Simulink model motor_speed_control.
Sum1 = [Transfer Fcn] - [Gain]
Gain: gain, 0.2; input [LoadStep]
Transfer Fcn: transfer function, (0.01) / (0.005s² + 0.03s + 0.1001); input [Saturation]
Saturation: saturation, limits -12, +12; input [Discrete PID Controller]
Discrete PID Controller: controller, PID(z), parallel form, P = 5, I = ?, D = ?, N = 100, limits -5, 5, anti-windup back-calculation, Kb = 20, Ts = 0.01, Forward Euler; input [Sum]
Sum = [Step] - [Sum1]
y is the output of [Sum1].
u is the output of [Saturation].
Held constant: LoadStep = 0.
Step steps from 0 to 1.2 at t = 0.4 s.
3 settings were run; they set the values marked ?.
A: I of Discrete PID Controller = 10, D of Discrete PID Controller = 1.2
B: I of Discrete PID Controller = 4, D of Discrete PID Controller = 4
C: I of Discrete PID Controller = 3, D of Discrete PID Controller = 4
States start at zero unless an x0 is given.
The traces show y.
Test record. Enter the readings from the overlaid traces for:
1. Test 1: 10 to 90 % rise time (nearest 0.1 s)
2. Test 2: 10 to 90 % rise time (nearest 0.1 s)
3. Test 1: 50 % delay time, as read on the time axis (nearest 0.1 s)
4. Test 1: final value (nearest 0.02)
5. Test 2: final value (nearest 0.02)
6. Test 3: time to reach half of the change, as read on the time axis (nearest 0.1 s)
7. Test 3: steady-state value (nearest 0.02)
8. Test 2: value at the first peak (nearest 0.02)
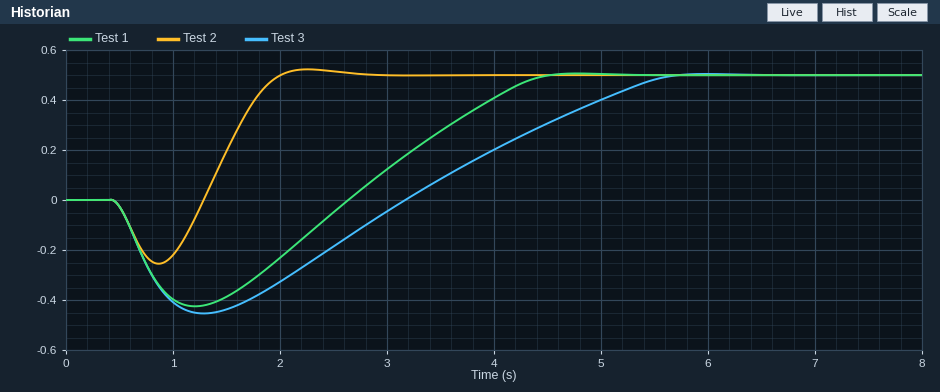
1.4 s
0.5 s
3.4 s
0.50
0.50
4.2 s
0.50
0.52
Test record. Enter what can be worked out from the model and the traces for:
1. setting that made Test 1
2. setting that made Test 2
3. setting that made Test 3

B
A
C
